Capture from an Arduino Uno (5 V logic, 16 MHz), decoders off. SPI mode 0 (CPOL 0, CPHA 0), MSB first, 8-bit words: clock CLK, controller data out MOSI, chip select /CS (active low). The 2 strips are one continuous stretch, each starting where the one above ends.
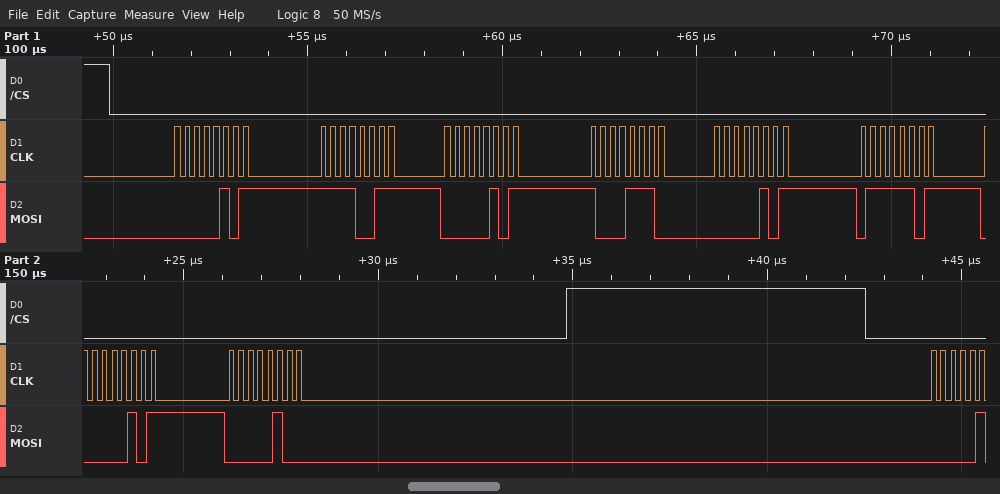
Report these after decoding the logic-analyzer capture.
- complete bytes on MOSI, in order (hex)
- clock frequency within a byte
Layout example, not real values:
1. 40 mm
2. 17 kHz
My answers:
1. 0x05 0xF3 0x05 0x8E 0x05 0x7D 0x05 0x04
2. 4 MHz
